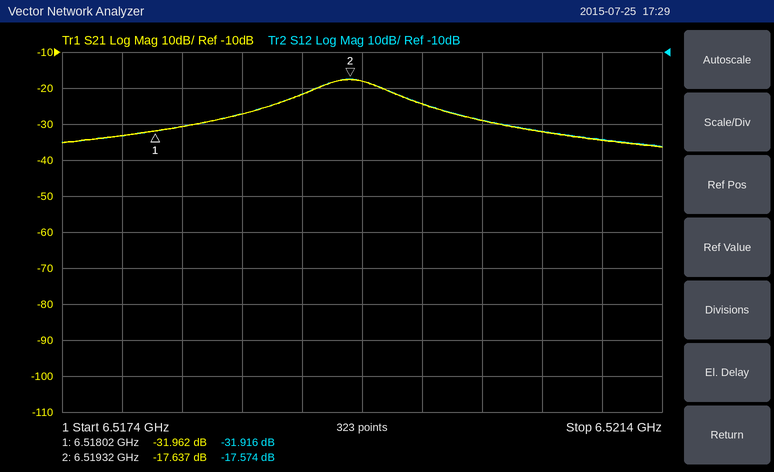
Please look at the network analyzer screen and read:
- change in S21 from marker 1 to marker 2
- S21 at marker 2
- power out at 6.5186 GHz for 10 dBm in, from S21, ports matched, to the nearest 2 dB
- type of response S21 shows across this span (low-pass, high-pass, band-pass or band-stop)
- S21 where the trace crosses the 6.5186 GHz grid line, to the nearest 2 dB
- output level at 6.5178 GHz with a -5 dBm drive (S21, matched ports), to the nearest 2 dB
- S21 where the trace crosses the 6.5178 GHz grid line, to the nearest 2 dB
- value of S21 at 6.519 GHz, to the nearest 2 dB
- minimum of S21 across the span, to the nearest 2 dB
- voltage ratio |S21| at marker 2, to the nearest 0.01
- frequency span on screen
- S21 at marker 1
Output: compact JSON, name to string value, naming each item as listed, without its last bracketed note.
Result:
{"change in S21 from marker 1 to marker 2": "14.325 dB", "S21 at marker 2": "-17.637 dB", "power out at 6.5186 GHz for 10 dBm in, from S21, ports matched, to the nearest 2 dB": "-18 dBm", "type of response S21 shows across this span": "band-pass", "S21 where the trace crosses the 6.5186 GHz grid line, to the nearest 2 dB": "-28 dB", "output level at 6.5178 GHz with a -5 dBm drive (S21, matched ports), to the nearest 2 dB": "-38 dBm", "S21 where the trace crosses the 6.5178 GHz grid line, to the nearest 2 dB": "-34 dB", "value of S21 at 6.519 GHz, to the nearest 2 dB": "-22 dB", "minimum of S21 across the span, to the nearest 2 dB": "-36 dB", "voltage ratio |S21| at marker 2, to the nearest 0.01": "0.13", "frequency span on screen": "4 MHz", "S21 at marker 1": "-31.962 dB"}
